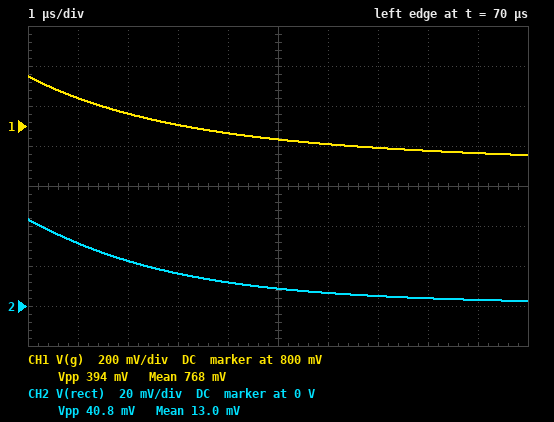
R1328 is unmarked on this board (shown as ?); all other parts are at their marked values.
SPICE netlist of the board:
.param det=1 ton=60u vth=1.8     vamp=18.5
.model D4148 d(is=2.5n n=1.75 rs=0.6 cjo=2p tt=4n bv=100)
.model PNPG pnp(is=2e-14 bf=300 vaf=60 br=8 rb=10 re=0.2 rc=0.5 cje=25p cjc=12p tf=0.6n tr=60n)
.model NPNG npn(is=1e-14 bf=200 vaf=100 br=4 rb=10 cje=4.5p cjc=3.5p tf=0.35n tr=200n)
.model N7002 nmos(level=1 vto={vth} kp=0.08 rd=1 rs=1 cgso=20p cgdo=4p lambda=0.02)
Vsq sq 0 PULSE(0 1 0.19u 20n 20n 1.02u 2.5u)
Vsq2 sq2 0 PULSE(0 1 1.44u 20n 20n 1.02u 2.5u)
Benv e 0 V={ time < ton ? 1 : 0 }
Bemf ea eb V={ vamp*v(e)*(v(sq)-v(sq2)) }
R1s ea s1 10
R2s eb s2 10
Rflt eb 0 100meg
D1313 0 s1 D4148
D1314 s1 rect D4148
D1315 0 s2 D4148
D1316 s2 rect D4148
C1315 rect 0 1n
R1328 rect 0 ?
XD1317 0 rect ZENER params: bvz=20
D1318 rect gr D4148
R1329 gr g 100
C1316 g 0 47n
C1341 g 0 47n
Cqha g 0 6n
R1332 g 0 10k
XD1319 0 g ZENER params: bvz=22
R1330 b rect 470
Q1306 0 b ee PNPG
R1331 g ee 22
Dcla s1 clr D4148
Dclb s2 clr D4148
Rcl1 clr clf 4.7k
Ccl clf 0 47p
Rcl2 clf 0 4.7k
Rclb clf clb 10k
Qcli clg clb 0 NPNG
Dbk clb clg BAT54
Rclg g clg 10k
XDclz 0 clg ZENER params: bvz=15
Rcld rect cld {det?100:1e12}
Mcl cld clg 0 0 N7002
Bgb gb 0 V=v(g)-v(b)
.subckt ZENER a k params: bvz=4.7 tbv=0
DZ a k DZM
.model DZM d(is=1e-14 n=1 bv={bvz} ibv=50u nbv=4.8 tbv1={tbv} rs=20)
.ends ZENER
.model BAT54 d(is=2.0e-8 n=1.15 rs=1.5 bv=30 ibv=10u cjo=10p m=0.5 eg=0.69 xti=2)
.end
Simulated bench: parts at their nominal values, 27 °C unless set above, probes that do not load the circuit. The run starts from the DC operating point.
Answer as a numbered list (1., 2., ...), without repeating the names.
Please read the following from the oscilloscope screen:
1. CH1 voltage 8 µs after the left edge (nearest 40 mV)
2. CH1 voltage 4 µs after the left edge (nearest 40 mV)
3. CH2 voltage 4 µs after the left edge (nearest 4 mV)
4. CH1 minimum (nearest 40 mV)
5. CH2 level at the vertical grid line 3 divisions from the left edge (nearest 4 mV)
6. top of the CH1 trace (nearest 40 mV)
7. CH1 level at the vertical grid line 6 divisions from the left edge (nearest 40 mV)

1. 680 mV
2. 760 mV
3. 12 mV
4. 640 mV
5. 16 mV
6. 1.04 V
7. 720 mV
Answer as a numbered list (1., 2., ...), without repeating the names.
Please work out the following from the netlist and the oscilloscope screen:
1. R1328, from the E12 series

1. 820 Ω
